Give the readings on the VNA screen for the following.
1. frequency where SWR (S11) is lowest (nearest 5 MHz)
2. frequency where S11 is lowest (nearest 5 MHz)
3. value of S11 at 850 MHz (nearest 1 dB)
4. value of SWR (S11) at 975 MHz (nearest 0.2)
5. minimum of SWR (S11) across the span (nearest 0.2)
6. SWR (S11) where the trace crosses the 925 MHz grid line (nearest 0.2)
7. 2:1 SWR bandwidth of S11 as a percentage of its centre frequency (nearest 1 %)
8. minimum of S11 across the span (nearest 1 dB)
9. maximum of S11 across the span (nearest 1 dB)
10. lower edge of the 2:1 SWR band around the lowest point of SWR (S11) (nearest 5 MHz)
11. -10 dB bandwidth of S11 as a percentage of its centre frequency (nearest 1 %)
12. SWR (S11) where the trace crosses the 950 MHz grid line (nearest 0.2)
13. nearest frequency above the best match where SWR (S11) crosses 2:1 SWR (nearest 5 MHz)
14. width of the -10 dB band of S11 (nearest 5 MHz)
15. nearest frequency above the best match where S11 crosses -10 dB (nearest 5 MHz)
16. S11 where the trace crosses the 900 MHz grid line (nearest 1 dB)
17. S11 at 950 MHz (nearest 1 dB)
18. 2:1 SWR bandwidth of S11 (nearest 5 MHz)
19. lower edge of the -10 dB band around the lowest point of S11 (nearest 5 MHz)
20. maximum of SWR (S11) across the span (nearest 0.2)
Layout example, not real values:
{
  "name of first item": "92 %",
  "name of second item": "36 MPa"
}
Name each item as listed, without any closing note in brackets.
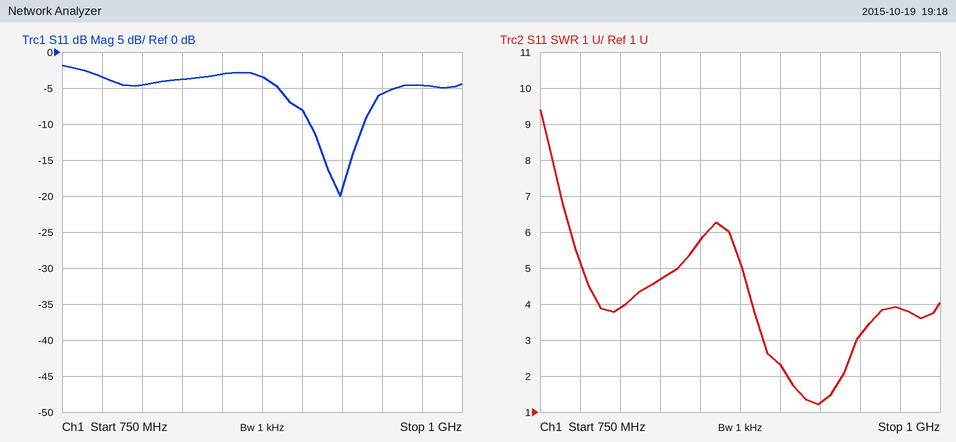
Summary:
{
  "frequency where SWR (S11) is lowest": "925 MHz",
  "frequency where S11 is lowest": "925 MHz",
  "value of S11 at 850 MHz": "-3 dB",
  "value of SWR (S11) at 975 MHz": "3.8",
  "minimum of SWR (S11) across the span": "1.2",
  "SWR (S11) where the trace crosses the 925 MHz grid line": "1.2",
  "2:1 SWR bandwidth of S11 as a percentage of its centre frequency": "4 %",
  "minimum of S11 across the span": "-20 dB",
  "maximum of S11 across the span": "-2 dB",
  "lower edge of the 2:1 SWR band around the lowest point of SWR (S11)": "905 MHz",
  "-10 dB bandwidth of S11 as a percentage of its centre frequency": "4 %",
  "SWR (S11) where the trace crosses the 950 MHz grid line": "3.2",
  "nearest frequency above the best match where SWR (S11) crosses 2:1 SWR": "940 MHz",
  "width of the -10 dB band of S11": "35 MHz",
  "nearest frequency above the best match where S11 crosses -10 dB": "940 MHz",
  "S11 where the trace crosses the 900 MHz grid line": "-8 dB",
  "S11 at 950 MHz": "-6 dB",
  "2:1 SWR bandwidth of S11": "35 MHz",
  "lower edge of the -10 dB band around the lowest point of S11": "905 MHz",
  "maximum of SWR (S11) across the span": "9.4"
}
